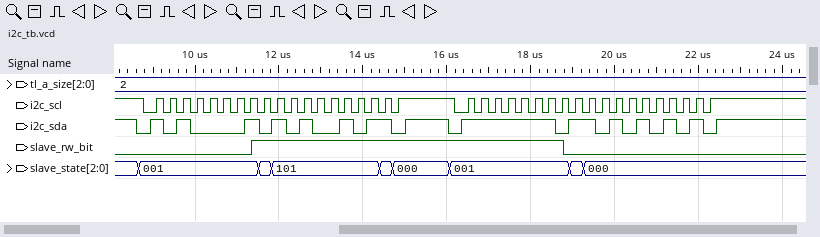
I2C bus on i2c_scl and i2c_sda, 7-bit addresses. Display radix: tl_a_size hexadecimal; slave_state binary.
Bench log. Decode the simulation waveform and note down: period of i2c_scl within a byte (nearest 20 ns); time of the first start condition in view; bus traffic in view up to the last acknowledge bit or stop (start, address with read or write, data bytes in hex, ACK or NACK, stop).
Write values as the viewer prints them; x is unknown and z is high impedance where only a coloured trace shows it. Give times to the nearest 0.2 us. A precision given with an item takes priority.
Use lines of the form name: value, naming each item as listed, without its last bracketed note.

period of i2c_scl within a byte: 320 ns
time of the first start condition in view: 8.6 us
bus traffic in view up to the last acknowledge bit or stop: start, address 50 read ACK, A5 NACK, stop, start, address 7F write NACK, AA NACK, stop
